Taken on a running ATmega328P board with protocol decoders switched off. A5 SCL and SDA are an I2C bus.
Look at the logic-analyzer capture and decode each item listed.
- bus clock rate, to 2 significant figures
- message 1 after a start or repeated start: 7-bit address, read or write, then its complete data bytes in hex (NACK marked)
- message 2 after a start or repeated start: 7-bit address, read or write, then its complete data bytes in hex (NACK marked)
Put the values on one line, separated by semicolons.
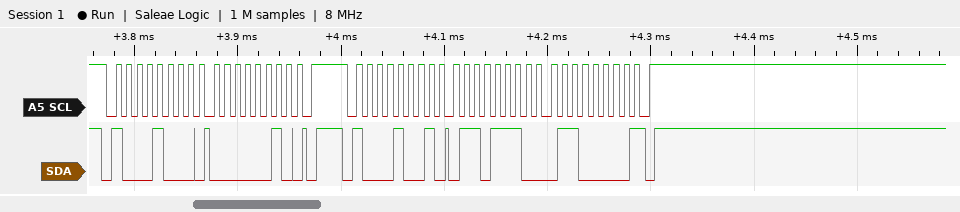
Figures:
100 kHz; 0x44 write: 02; 0x44 read: 6E 60 NACK
